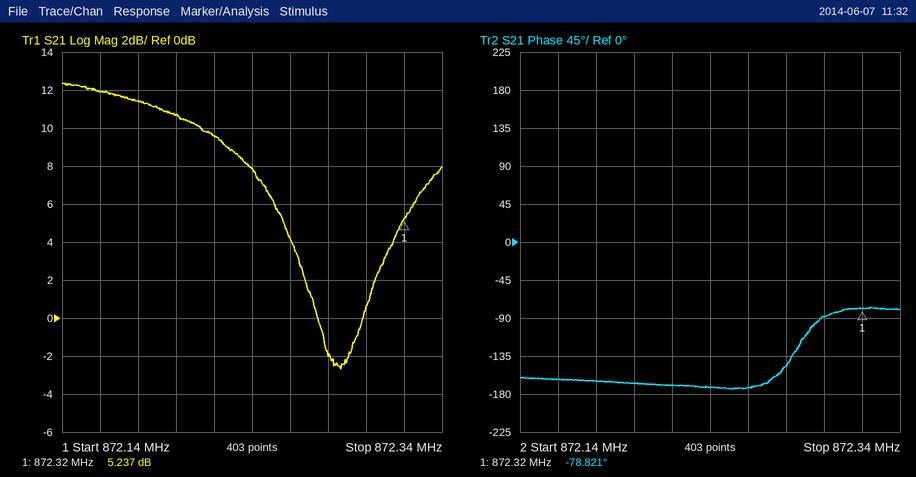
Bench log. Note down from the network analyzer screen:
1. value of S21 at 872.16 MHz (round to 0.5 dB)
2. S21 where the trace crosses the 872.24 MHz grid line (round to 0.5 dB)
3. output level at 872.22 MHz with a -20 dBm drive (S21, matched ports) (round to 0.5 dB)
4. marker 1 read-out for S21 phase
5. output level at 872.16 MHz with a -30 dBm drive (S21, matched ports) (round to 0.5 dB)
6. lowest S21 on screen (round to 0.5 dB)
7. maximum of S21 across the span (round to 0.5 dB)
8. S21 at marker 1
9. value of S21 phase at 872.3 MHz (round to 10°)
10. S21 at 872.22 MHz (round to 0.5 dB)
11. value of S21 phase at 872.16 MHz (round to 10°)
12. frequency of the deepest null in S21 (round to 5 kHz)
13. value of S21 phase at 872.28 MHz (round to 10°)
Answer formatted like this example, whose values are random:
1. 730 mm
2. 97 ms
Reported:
1. 12.0 dB
2. 8.0 dB
3. -10.5 dBm
4. -78.821°
5. -18.0 dBm
6. -2.5 dB
7. 12.5 dB
8. 5.237 dB
9. -90°
10. 9.5 dB
11. -160°
12. 872.285 MHz
13. -150°
